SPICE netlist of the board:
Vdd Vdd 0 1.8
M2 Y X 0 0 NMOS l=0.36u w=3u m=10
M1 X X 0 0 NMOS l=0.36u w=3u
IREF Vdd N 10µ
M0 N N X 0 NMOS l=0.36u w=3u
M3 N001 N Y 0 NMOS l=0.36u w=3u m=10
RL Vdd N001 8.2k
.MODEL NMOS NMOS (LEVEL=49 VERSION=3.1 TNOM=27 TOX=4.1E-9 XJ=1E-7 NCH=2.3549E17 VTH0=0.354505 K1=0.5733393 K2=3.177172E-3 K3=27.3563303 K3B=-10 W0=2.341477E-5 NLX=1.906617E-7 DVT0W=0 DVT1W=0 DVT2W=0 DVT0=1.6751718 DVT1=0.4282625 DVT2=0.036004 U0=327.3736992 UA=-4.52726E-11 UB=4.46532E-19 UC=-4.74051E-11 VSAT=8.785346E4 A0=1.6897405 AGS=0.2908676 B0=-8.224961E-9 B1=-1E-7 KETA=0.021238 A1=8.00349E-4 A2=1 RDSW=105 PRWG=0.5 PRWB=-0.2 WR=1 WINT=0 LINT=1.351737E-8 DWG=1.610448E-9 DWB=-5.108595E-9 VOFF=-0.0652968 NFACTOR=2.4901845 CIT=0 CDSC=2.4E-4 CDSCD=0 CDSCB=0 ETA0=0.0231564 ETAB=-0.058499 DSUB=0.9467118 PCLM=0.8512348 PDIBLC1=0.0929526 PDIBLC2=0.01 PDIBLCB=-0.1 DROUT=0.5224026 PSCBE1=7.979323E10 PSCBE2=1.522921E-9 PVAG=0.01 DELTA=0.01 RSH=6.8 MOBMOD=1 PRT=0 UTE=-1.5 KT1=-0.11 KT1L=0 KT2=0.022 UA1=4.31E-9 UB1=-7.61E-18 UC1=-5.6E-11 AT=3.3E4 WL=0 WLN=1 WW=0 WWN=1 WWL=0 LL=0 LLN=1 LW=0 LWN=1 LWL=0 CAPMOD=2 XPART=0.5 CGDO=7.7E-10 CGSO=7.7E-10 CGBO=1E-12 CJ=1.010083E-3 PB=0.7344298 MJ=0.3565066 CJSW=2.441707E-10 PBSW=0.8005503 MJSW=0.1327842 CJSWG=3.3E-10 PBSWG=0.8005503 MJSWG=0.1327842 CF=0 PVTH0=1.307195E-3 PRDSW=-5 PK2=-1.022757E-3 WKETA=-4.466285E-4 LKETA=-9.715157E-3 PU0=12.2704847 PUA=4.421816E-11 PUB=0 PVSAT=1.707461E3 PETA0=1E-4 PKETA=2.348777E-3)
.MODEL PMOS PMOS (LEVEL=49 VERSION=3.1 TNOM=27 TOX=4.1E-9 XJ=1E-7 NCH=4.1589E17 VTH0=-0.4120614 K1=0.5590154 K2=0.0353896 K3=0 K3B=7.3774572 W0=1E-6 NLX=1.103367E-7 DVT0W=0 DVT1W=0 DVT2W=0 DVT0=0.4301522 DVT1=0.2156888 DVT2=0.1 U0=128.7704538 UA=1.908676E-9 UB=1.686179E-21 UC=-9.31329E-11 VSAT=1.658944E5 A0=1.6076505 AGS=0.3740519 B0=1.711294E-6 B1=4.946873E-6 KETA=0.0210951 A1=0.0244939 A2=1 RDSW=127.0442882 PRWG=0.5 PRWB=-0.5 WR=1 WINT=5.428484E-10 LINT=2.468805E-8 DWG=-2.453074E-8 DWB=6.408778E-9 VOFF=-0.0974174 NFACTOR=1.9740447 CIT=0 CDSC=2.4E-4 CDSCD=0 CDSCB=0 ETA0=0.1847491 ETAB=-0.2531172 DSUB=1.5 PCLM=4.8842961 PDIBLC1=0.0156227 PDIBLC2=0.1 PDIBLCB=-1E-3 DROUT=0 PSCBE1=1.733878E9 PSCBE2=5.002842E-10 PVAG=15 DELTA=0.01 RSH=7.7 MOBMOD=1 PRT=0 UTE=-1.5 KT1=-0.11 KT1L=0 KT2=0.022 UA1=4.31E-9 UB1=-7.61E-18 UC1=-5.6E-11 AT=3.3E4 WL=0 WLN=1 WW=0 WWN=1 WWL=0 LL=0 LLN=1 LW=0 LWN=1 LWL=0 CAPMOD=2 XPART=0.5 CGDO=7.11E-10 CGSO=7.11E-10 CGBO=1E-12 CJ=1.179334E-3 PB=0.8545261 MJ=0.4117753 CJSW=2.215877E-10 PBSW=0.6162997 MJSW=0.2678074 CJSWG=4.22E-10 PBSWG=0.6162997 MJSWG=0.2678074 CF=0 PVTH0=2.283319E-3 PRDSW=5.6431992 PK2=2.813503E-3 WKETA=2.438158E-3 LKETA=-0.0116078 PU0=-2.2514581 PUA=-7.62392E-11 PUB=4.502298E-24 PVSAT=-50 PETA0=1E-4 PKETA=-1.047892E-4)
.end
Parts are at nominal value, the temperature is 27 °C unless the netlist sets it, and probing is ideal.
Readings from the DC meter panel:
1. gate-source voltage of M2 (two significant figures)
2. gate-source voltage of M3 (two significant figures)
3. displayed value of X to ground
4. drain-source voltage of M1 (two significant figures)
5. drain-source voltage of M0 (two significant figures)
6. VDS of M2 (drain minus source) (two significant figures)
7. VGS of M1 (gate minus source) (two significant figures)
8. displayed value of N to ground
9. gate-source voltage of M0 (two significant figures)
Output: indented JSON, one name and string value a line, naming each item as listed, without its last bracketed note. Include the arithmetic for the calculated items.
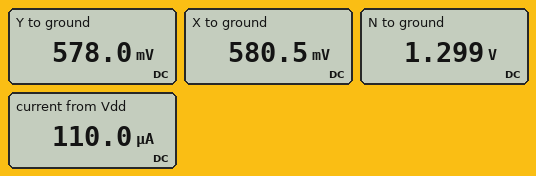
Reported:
{
  "gate-source voltage of M2": "580.5 mV = 580 mV",
  "gate-source voltage of M3": "1.299 V - 578 mV = 720 mV",
  "displayed value of X to ground": "580.5 mV",
  "drain-source voltage of M1": "580.5 mV = 580 mV",
  "drain-source voltage of M0": "1.299 V - 580.5 mV = 720 mV",
  "VDS of M2 (drain minus source)": "578 mV = 580 mV",
  "VGS of M1 (gate minus source)": "580.5 mV = 580 mV",
  "displayed value of N to ground": "1.299 V",
  "gate-source voltage of M0": "1.299 V - 580.5 mV = 720 mV"
}
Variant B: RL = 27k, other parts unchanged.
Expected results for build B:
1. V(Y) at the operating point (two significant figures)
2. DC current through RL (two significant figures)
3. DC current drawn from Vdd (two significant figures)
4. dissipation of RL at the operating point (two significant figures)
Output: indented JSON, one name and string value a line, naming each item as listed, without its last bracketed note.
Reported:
{
  "V(Y) at the operating point": "53 mV",
  "DC current through RL": "65 µA",
  "DC current drawn from Vdd": "75 µA",
  "dissipation of RL at the operating point": "110 µW"
}
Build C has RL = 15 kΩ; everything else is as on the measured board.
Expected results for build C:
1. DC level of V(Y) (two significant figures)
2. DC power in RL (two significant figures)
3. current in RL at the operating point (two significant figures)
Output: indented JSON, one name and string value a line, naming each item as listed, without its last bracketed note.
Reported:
{
  "DC level of V(Y)": "350 mV",
  "DC power in RL": "140 µW",
  "current in RL at the operating point": "96 µA"
}
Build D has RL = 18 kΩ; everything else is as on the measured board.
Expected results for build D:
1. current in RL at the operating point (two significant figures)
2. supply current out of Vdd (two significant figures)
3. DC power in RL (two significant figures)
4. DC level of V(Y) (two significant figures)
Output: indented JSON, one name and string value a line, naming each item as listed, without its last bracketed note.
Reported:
{
  "current in RL at the operating point": "91 µA",
  "supply current out of Vdd": "100 µA",
  "DC power in RL": "150 µW",
  "DC level of V(Y)": "160 mV"
}
